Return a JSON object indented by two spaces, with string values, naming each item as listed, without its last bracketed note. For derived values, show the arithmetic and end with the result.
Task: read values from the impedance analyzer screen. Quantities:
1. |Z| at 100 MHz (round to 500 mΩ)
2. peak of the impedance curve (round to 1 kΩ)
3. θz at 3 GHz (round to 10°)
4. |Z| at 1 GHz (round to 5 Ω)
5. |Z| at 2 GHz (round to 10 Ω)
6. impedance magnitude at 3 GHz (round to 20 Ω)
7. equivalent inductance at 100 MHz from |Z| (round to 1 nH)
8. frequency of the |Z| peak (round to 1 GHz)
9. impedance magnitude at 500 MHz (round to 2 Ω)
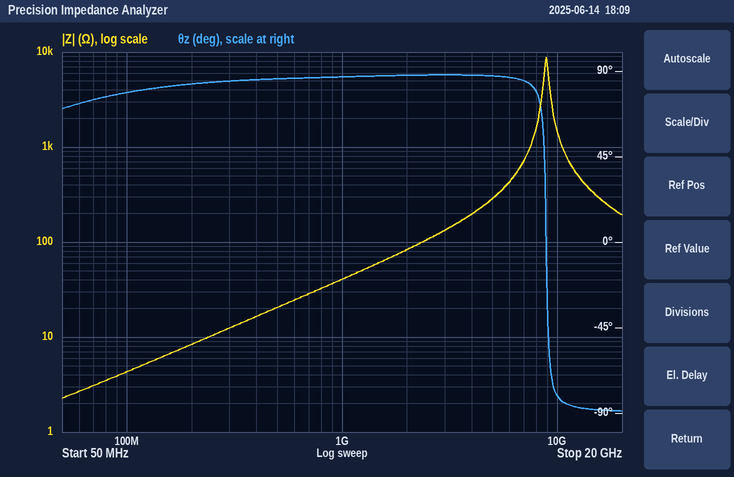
{
  "|Z| at 100 MHz": "4.5 Ω",
  "peak of the impedance curve": "9 kΩ",
  "θz at 3 GHz": "90°",
  "|Z| at 1 GHz": "40 Ω",
  "|Z| at 2 GHz": "80 Ω",
  "impedance magnitude at 3 GHz": "140 Ω",
  "equivalent inductance at 100 MHz from |Z|": "L = 4.5 Ω/(2π × 100 MHz) ≈ 7 nH",
  "frequency of the |Z| peak": "9 GHz",
  "impedance magnitude at 500 MHz": "20 Ω"
}
